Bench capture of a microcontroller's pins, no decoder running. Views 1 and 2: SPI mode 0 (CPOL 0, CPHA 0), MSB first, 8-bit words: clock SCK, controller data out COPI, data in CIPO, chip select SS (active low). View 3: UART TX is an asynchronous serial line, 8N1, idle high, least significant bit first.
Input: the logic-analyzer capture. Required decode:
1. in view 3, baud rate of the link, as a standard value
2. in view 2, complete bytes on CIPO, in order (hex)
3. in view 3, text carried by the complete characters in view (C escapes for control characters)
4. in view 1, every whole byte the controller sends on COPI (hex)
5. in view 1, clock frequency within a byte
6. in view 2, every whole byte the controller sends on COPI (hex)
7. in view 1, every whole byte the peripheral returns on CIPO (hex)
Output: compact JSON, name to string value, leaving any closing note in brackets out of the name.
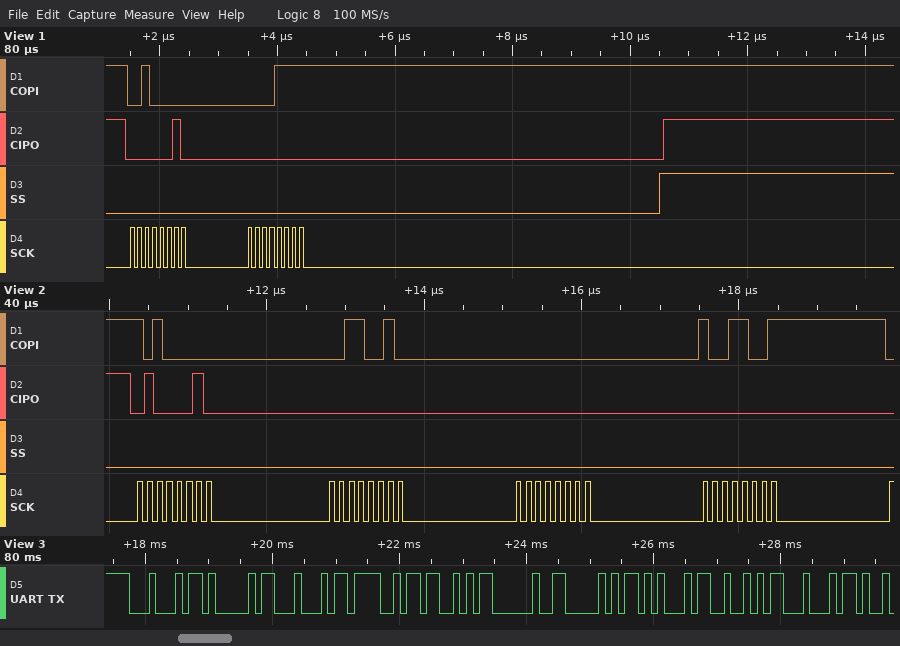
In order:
{"in view 3, baud rate of the link, as a standard value": "9600 baud", "in view 2, complete bytes on CIPO, in order": "42 00 00 00", "in view 3, text carried by the complete characters in view": "\"DADOS PERD\"", "in view 1, every whole byte the controller sends on COPI": "0x20 0x0F", "in view 1, clock frequency within a byte": "8 MHz", "in view 2, every whole byte the controller sends on COPI": "A0 32 00 99", "in view 1, every whole byte the peripheral returns on CIPO": "0x02 0x00"}
